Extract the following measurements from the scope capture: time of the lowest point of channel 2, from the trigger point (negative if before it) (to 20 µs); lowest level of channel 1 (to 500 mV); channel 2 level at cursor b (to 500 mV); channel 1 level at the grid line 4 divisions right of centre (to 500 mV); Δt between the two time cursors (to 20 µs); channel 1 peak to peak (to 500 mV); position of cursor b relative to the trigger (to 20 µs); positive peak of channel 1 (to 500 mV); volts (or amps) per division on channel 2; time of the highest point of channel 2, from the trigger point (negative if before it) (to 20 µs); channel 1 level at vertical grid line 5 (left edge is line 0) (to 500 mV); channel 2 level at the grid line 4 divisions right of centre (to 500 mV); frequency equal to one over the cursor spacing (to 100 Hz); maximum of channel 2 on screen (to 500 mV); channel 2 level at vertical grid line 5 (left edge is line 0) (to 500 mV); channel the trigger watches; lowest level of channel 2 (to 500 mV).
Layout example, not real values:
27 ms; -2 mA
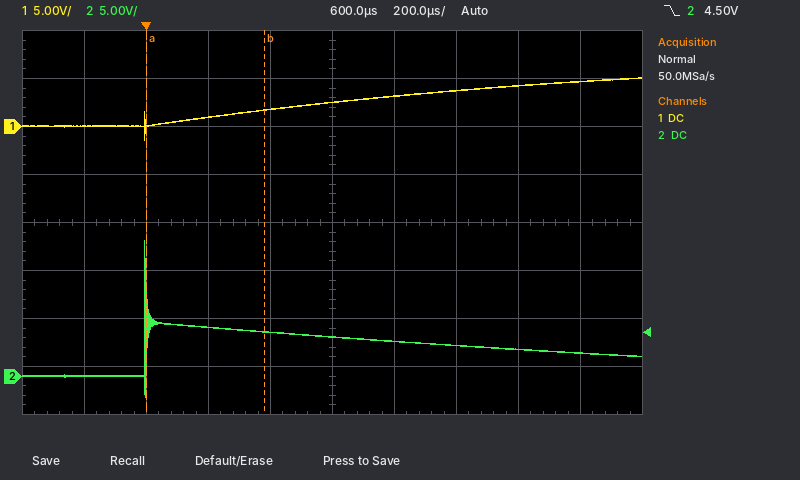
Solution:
0 µs; -1.5 V; 4.5 V; 4.5 V; 380 µs; 6.5 V; +380 µs; 5.0 V; 5 V; 0 µs; 2.5 V; 2.5 V; 2.6 kHz; 14.0 V; 4.0 V; channel 2; -2.0 V
